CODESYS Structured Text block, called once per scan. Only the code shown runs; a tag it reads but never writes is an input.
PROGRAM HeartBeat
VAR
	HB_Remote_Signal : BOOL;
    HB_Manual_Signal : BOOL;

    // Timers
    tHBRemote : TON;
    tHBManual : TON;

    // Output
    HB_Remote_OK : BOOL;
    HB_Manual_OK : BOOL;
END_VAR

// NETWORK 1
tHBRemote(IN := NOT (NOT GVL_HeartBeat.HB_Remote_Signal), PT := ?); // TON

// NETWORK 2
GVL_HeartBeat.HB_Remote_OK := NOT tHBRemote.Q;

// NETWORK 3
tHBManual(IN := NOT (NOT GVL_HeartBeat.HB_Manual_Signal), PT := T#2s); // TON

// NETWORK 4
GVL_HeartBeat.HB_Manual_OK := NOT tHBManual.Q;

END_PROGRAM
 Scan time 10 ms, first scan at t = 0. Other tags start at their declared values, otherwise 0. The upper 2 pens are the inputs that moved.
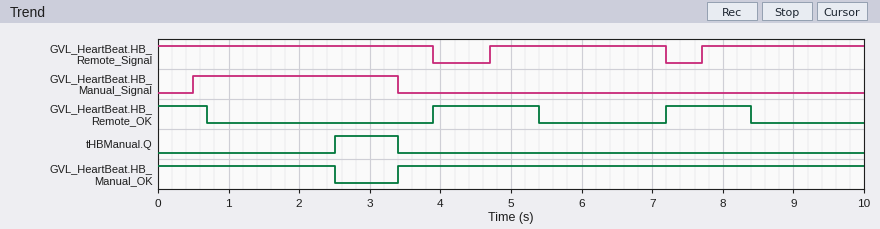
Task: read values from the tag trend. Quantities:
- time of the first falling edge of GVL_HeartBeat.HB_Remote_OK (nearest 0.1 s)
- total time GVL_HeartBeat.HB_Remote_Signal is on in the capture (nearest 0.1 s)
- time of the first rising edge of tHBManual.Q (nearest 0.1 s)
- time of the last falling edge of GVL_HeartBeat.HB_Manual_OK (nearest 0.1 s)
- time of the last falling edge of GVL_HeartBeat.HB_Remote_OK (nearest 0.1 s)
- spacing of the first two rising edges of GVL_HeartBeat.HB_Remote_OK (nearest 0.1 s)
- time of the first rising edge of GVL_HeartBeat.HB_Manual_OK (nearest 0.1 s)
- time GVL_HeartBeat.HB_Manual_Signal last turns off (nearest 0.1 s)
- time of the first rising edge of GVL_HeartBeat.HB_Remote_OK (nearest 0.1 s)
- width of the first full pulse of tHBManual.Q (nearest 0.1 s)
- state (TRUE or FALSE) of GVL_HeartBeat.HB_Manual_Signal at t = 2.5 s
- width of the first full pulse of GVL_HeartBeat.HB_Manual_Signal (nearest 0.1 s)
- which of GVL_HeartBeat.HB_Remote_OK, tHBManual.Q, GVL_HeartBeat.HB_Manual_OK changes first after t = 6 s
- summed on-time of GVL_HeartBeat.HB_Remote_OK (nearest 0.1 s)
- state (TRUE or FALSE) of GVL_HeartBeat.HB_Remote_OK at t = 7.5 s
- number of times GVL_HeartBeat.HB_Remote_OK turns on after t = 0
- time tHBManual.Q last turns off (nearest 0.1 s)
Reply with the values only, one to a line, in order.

0.7 s
8.7 s
2.5 s
2.5 s
8.4 s
3.3 s
3.4 s
3.4 s
3.9 s
0.9 s
TRUE
2.9 s
GVL_HeartBeat.HB_Remote_OK
3.4 s
TRUE
2
3.4 s
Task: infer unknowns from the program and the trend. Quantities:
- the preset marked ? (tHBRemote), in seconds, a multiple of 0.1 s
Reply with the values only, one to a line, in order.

0.7 s
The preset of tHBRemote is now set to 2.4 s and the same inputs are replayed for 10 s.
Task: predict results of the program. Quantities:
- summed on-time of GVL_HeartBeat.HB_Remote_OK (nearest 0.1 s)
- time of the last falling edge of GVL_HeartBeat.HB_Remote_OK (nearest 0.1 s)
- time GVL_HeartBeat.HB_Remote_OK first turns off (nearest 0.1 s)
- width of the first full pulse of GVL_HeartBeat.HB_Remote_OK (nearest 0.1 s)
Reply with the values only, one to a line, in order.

8.4 s
7.1 s
2.4 s
3.2 s
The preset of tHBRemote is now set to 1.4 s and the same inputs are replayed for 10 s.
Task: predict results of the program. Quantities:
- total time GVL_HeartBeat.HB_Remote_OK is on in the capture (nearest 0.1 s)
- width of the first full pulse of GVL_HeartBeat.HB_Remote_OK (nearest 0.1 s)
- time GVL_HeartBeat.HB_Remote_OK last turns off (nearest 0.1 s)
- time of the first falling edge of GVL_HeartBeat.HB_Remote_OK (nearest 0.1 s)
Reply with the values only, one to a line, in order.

5.5 s
2.2 s
9.1 s
1.4 s
